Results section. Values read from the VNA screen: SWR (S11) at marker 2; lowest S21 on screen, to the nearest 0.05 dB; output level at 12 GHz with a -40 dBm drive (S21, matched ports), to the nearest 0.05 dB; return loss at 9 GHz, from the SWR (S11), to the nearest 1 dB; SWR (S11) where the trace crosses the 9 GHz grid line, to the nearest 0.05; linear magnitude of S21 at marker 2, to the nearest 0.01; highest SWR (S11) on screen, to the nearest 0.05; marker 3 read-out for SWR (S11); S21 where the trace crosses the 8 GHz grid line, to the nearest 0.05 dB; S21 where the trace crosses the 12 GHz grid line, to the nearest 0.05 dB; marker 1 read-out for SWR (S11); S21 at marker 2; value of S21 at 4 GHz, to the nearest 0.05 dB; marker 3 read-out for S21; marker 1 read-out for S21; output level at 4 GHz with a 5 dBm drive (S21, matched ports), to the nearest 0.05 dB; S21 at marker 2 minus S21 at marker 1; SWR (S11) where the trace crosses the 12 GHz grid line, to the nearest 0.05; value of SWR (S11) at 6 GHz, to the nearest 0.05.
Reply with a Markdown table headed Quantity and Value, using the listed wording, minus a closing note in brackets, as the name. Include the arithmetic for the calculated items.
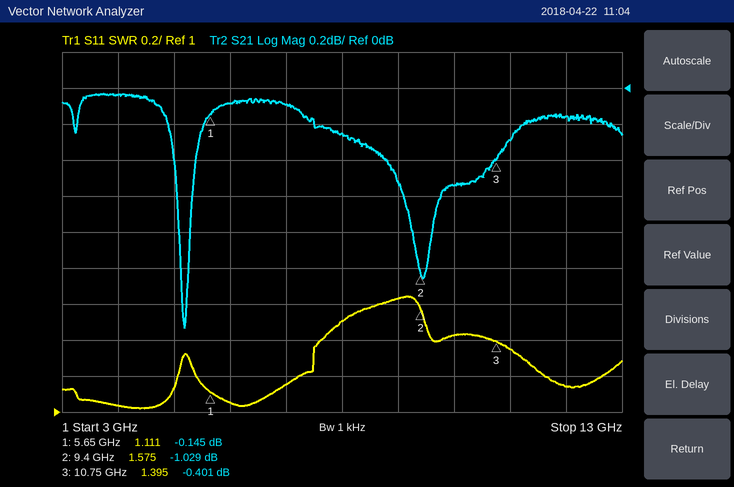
| Quantity | Value |
|---|---|
| SWR (S11) at marker 2 | 1.575 |
| lowest S21 on screen, to the nearest 0.05 dB | -1.35 dB |
| output level at 12 GHz with a -40 dBm drive (S21, matched ports), to the nearest 0.05 dB | -40 dBm + (-0.15 dB) = -40.15 dBm |
| return loss at 9 GHz, from the SWR (S11), to the nearest 1 dB | −20 log10((1.65 − 1)/(1.65 + 1)) ≈ 12 dB |
| SWR (S11) where the trace crosses the 9 GHz grid line, to the nearest 0.05 | 1.65 |
| linear magnitude of S21 at marker 2, to the nearest 0.01 | 10^(-1.029/20) ≈ 0.89 |
| highest SWR (S11) on screen, to the nearest 0.05 | 1.65 |
| marker 3 read-out for SWR | 1.395 |
| S21 where the trace crosses the 8 GHz grid line, to the nearest 0.05 dB | -0.25 dB |
| S21 where the trace crosses the 12 GHz grid line, to the nearest 0.05 dB | -0.15 dB |
| marker 1 read-out for SWR | 1.111 |
| S21 at marker 2 | -1.029 dB |
| value of S21 at 4 GHz, to the nearest 0.05 dB | -0.05 dB |
| marker 3 read-out for S21 | -0.401 dB |
| marker 1 read-out for S21 | -0.145 dB |
| output level at 4 GHz with a 5 dBm drive (S21, matched ports), to the nearest 0.05 dB | 5 dBm + (-0.05 dB) = 4.95 dBm |
| S21 at marker 2 minus S21 at marker 1 | -1.029 − (-0.145) = -0.884 dB |
| SWR (S11) where the trace crosses the 12 GHz grid line, to the nearest 0.05 | 1.15 |
| value of SWR (S11) at 6 GHz, to the nearest 0.05 | 1.05 |
